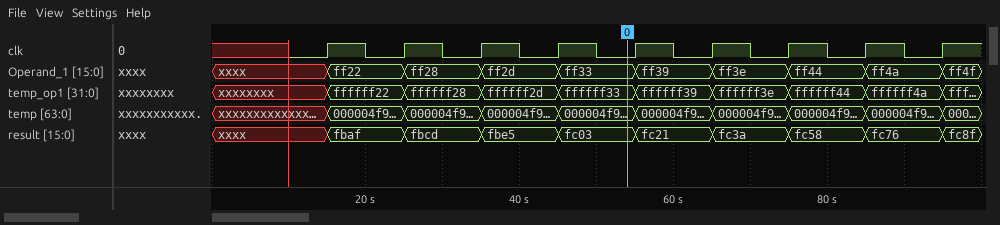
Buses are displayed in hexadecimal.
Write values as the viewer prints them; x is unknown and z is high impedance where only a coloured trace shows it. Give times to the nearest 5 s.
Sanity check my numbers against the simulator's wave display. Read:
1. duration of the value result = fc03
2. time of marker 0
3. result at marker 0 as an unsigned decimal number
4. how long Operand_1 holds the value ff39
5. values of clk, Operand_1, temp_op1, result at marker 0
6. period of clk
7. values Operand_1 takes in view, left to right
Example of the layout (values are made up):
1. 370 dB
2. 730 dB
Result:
1. 10 s
2. 55 s
3. 64515
4. 10 s
5. clk=0, Operand_1=ff33, temp_op1=ffffff33, result=fc03
6. 10 s
7. xxxx, ff22, ff28, ff2d, ff33, ff39, ff3e, ff44, ff4a, ff4f
